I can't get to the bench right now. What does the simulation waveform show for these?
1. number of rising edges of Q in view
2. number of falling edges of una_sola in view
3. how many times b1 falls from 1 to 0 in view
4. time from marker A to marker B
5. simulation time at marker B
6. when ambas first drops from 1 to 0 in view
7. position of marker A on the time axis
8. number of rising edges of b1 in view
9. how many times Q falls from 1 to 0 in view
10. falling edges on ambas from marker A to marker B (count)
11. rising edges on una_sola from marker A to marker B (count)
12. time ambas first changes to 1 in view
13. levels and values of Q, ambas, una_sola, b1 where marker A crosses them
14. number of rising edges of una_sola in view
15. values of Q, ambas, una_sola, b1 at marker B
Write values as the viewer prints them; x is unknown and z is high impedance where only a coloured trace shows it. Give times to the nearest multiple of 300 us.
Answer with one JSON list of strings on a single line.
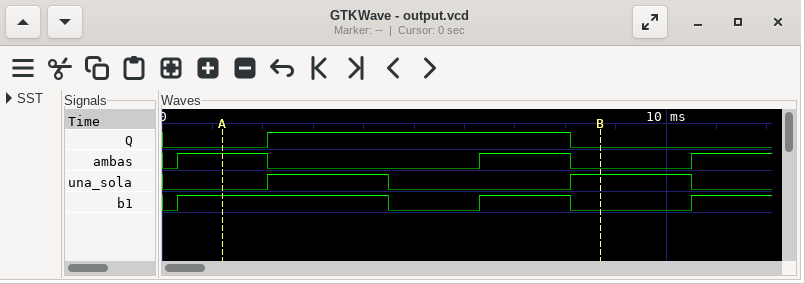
["1", "2", "2", "7500 us", "8700 us", "2100 us", "1200 us", "3", "1", "2", "2", "300 us", "Q=0, ambas=1, una_sola=0, b1=1", "2", "Q=0, ambas=0, una_sola=1, b1=0"]
